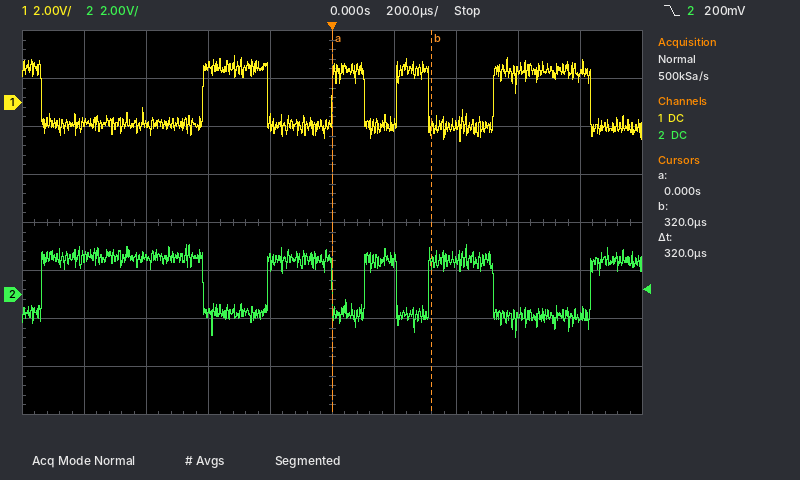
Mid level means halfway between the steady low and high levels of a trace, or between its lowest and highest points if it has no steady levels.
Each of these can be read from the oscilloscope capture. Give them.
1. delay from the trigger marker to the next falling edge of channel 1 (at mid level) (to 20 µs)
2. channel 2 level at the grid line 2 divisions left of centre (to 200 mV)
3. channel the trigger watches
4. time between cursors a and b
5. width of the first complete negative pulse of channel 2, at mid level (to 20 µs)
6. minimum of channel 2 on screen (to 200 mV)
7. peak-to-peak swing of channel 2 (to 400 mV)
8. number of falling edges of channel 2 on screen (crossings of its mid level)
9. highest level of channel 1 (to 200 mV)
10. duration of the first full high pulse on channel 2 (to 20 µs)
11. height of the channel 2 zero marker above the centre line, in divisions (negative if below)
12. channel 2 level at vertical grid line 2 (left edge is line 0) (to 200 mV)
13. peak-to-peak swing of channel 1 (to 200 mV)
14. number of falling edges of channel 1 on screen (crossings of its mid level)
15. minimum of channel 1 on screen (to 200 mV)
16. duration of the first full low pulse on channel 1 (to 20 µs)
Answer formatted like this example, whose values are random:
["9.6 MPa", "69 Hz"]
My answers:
["100 µs", "-800 mV", "channel 2", "320 µs", "200 µs", "-1.8 V", "4.0 V", "4", "2.0 V", "520 µs", "-1.5 div", "1.6 V", "3.6 V", "5", "-1.6 V", "520 µs"]
